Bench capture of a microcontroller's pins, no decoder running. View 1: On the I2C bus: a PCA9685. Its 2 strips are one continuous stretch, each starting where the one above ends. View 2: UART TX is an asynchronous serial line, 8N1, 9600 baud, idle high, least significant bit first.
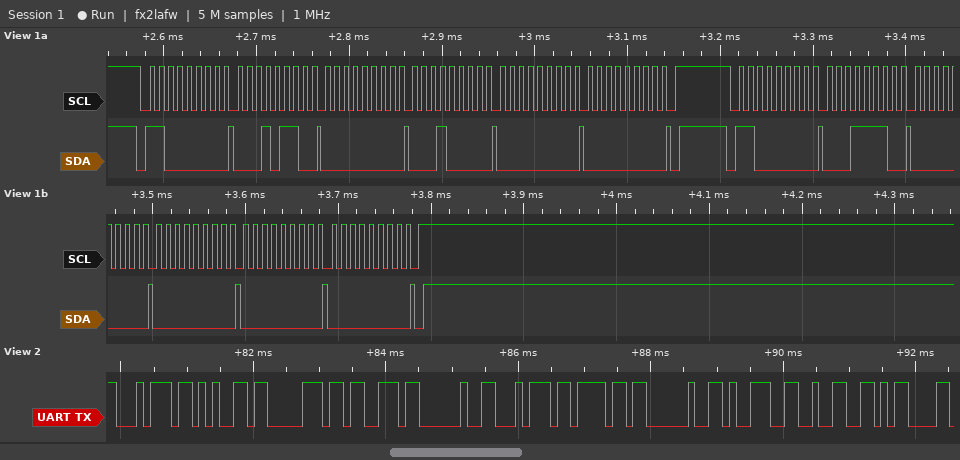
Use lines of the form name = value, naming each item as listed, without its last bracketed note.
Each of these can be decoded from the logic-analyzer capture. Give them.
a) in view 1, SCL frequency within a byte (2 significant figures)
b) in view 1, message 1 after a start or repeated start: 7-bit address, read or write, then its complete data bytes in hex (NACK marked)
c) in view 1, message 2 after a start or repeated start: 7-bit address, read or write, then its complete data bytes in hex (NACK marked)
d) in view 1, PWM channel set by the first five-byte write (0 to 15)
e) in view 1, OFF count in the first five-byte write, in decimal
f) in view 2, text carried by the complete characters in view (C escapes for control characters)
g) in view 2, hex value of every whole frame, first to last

in view 1, SCL frequency within a byte = 100 kHz
in view 1, message 1 after a start or repeated start: 7-bit address, read or write, then its complete data bytes in hex = 0x60 write: 16 00 10 00 00
in view 1, message 2 after a start or repeated start: 7-bit address, read or write, then its complete data bytes in hex = 0x60 write: 1E 00 00 00 00
in view 1, PWM channel set by the first five-byte write = 4
in view 1, OFF count in the first five-byte write, in decimal = 0
in view 2, text carried by the complete characters in view = "teps to 92\r"
in view 2, hex value of every whole frame, first to last = 74 65 70 73 20 74 6F 20 39 32 0D
